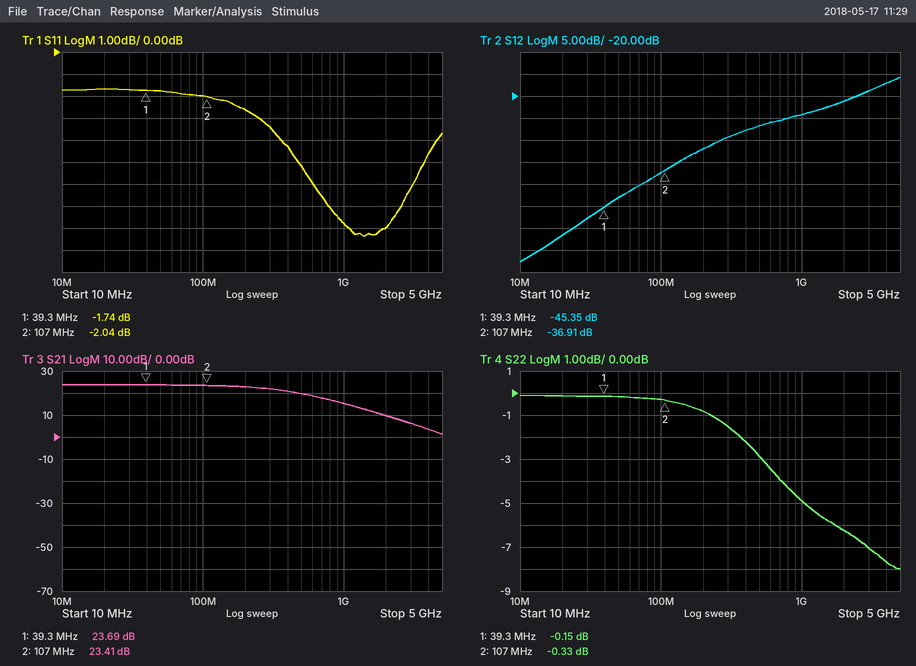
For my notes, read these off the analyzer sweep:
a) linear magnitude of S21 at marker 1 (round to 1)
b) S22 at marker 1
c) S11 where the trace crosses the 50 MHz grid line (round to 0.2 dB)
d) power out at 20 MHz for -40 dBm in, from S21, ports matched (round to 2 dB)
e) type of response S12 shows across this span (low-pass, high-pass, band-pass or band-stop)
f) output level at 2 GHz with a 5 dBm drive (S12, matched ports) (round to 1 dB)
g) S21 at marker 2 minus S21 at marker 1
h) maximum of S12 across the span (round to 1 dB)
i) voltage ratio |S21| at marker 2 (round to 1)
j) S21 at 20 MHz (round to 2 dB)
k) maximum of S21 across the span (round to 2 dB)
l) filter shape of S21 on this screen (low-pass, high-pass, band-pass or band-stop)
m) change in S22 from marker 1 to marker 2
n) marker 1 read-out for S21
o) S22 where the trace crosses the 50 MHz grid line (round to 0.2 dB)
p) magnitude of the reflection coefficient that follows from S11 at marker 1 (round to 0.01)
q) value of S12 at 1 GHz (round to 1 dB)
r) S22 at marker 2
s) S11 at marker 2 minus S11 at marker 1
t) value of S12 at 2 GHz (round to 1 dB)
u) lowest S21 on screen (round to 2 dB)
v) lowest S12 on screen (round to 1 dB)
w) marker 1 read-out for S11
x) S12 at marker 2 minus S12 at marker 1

15
-0.15 dB
-1.8 dB
-16 dBm
high-pass
-16 dBm
-0.28 dB
-16 dB
15
24 dB
24 dB
low-pass
-0.18 dB
23.69 dB
-0.2 dB
0.82
-24 dB
-0.33 dB
-0.30 dB
-21 dB
2 dB
-58 dB
-1.74 dB
8.44 dB
